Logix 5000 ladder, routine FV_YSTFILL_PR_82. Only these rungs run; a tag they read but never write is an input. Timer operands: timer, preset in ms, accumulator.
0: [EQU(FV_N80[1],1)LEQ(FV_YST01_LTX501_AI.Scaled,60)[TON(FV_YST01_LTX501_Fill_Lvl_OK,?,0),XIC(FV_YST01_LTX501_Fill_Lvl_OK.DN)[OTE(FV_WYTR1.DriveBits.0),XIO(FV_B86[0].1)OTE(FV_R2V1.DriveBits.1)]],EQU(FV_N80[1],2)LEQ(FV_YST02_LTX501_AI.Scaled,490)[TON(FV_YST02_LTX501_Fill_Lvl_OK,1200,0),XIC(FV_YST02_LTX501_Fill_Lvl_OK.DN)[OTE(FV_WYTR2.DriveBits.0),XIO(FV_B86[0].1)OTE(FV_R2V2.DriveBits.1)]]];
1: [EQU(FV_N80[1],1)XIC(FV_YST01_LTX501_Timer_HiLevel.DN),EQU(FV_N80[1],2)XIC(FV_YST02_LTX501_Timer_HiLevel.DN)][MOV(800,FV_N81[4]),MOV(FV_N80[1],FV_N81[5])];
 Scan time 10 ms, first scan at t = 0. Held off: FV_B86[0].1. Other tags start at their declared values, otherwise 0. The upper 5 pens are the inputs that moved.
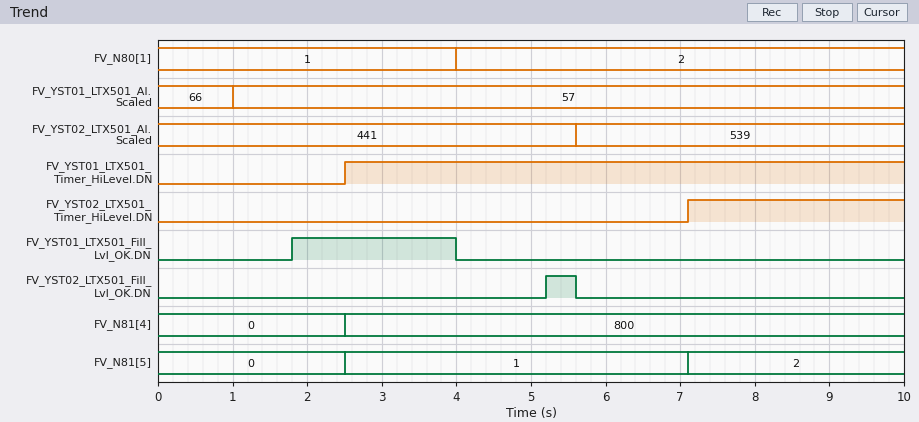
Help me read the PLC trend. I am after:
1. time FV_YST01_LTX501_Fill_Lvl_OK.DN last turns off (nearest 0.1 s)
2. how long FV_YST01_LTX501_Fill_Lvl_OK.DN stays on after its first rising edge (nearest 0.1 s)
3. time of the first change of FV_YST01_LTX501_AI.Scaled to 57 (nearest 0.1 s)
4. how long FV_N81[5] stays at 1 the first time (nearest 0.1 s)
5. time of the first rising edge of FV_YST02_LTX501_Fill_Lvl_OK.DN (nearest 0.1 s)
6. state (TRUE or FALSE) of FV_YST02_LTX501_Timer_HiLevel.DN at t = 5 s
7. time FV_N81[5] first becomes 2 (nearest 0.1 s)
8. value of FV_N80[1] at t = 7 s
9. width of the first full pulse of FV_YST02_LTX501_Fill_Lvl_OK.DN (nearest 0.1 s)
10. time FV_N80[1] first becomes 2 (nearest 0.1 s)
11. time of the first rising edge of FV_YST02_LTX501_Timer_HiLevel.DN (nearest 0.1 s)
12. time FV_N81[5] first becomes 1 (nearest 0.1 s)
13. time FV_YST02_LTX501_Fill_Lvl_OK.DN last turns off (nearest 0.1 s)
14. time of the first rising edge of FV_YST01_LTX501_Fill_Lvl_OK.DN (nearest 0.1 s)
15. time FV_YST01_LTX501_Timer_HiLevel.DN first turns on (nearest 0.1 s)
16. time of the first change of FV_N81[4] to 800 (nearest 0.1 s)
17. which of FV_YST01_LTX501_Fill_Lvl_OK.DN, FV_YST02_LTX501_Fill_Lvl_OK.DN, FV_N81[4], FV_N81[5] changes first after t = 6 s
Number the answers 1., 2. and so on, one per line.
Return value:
1. 4.0 s
2. 2.2 s
3. 1.0 s
4. 4.6 s
5. 5.2 s
6. FALSE
7. 7.1 s
8. 2
9. 0.4 s
10. 4.0 s
11. 7.1 s
12. 2.5 s
13. 5.6 s
14. 1.8 s
15. 2.5 s
16. 2.5 s
17. FV_N81[5]
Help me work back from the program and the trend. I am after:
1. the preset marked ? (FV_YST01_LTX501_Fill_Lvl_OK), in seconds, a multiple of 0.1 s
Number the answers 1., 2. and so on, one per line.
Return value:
1. 0.8 s
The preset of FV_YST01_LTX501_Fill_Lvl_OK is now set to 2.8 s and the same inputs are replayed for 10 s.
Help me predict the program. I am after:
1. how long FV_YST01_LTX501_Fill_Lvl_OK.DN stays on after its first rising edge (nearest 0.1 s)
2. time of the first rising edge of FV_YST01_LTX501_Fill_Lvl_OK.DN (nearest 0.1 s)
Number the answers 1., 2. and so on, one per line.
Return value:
1. 0.2 s
2. 3.8 s
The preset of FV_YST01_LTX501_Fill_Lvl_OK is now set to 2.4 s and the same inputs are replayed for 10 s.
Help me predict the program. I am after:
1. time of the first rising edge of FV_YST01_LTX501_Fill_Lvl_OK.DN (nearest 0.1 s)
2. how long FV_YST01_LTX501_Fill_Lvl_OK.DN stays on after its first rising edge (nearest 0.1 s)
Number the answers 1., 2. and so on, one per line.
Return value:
1. 3.4 s
2. 0.6 s
